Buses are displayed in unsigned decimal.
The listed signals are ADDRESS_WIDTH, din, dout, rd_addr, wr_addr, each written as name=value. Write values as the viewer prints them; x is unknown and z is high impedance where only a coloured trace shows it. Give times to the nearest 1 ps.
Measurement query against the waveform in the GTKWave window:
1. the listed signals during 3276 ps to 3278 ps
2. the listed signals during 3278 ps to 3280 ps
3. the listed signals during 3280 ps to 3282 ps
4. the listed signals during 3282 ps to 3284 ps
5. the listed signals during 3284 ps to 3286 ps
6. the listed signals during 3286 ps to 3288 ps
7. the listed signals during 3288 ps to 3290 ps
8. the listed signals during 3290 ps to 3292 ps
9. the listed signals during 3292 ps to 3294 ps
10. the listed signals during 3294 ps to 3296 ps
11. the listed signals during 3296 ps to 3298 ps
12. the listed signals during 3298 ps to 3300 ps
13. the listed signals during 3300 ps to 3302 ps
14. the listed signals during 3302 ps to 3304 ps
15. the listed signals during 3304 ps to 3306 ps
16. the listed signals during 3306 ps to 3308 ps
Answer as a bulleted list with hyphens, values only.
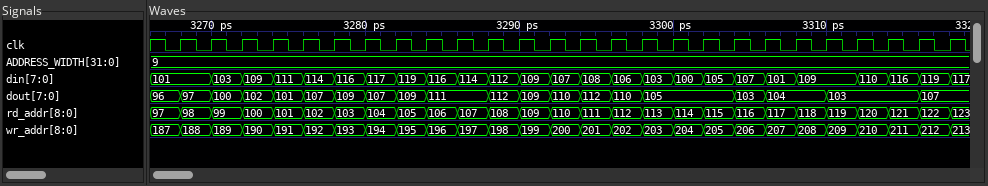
- ADDRESS_WIDTH=9, din=114, dout=107, rd_addr=102, wr_addr=192
- ADDRESS_WIDTH=9, din=116, dout=109, rd_addr=103, wr_addr=193
- ADDRESS_WIDTH=9, din=117, dout=107, rd_addr=104, wr_addr=194
- ADDRESS_WIDTH=9, din=119, dout=109, rd_addr=105, wr_addr=195
- ADDRESS_WIDTH=9, din=116, dout=111, rd_addr=106, wr_addr=196
- ADDRESS_WIDTH=9, din=114, dout=111, rd_addr=107, wr_addr=197
- ADDRESS_WIDTH=9, din=112, dout=112, rd_addr=108, wr_addr=198
- ADDRESS_WIDTH=9, din=109, dout=109, rd_addr=109, wr_addr=199
- ADDRESS_WIDTH=9, din=107, dout=110, rd_addr=110, wr_addr=200
- ADDRESS_WIDTH=9, din=108, dout=112, rd_addr=111, wr_addr=201
- ADDRESS_WIDTH=9, din=106, dout=110, rd_addr=112, wr_addr=202
- ADDRESS_WIDTH=9, din=103, dout=105, rd_addr=113, wr_addr=203
- ADDRESS_WIDTH=9, din=100, dout=105, rd_addr=114, wr_addr=204
- ADDRESS_WIDTH=9, din=105, dout=105, rd_addr=115, wr_addr=205
- ADDRESS_WIDTH=9, din=107, dout=103, rd_addr=116, wr_addr=206
- ADDRESS_WIDTH=9, din=101, dout=104, rd_addr=117, wr_addr=207
